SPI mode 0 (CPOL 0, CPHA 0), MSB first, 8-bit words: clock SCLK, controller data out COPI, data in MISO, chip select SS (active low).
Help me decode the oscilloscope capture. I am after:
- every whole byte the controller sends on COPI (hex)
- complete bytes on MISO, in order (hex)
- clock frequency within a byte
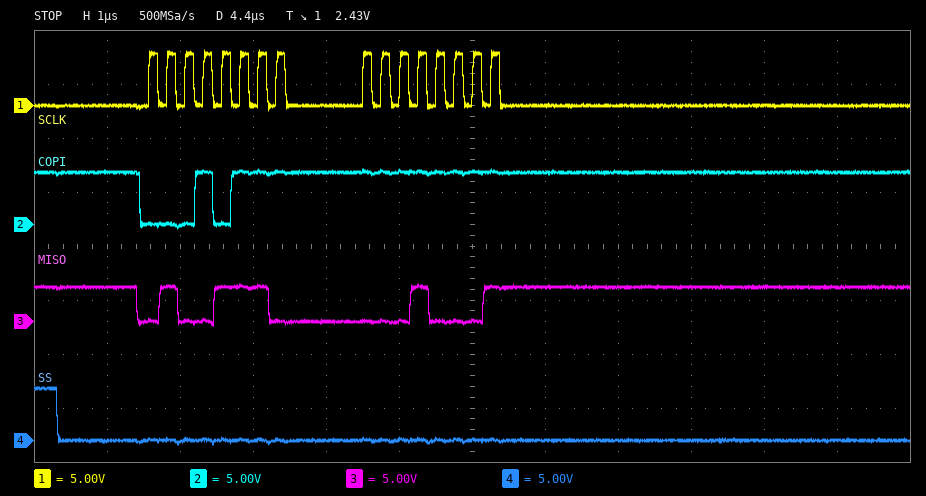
0x17 0xFF
0x4E 0x11
4 MHz
